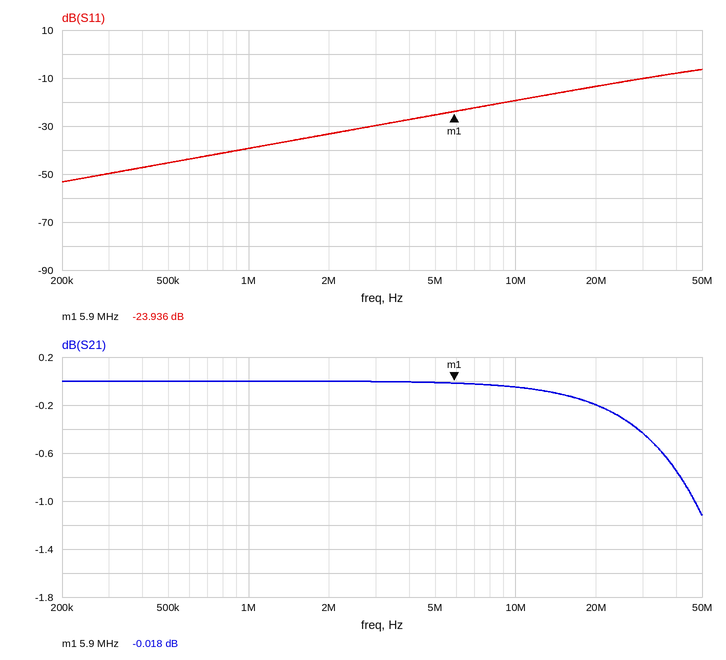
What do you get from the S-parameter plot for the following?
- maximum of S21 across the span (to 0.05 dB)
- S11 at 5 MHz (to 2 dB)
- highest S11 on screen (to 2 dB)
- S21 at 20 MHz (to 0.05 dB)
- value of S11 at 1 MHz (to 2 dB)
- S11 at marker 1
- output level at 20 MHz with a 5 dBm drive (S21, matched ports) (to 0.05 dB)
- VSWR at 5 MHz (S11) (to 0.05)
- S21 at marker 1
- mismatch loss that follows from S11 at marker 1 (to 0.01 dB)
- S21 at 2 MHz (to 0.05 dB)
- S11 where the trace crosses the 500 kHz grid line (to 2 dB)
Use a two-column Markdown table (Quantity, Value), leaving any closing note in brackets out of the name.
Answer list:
| Quantity | Value |
|---|---|
| maximum of S21 across the span | 0.00 dB |
| S11 at 5 MHz | -26 dB |
| highest S11 on screen | -6 dB |
| S21 at 20 MHz | -0.20 dB |
| value of S11 at 1 MHz | -40 dB |
| S11 at marker 1 | -23.936 dB |
| output level at 20 MHz with a 5 dBm drive (S21, matched ports) | 4.80 dBm |
| VSWR at 5 MHz (S11) | 1.10 |
| S21 at marker 1 | -0.018 dB |
| mismatch loss that follows from S11 at marker 1 | 0.02 dB |
| S21 at 2 MHz | 0.00 dB |
| S11 where the trace crosses the 500 kHz grid line | -46 dB |
